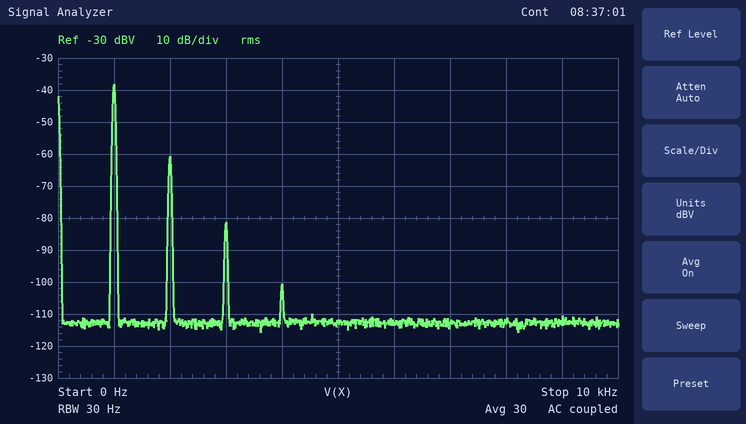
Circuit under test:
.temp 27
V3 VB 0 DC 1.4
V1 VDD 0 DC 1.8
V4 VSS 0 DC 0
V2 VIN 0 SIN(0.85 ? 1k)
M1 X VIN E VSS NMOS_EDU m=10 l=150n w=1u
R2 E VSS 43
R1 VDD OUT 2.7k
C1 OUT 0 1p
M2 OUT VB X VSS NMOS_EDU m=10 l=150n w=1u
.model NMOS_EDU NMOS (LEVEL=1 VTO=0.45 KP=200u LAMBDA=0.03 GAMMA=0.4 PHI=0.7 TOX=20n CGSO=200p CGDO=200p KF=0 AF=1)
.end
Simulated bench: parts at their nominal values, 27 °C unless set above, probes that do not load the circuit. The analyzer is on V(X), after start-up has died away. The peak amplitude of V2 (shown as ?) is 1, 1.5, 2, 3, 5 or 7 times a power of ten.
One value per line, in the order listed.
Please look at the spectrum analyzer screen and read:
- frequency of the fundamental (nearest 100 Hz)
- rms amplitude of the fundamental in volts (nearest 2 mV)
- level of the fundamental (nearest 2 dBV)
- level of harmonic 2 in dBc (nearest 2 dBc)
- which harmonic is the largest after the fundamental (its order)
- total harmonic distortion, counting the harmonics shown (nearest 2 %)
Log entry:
1.0 kHz
12 mV
-38 dBV
-22 dBc
2
8 %
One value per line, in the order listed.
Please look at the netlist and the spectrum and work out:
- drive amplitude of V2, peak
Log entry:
30 mV
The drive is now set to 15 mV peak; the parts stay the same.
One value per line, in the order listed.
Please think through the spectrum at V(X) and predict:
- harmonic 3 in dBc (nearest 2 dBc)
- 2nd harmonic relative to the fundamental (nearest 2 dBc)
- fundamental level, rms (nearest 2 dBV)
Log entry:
-56 dBc
-28 dBc
-44 dBV
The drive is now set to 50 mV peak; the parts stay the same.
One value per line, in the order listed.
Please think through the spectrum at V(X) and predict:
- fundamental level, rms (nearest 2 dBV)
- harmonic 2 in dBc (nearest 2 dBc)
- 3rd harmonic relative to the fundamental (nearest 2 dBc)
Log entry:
-34 dBV
-18 dBc
-34 dBc
